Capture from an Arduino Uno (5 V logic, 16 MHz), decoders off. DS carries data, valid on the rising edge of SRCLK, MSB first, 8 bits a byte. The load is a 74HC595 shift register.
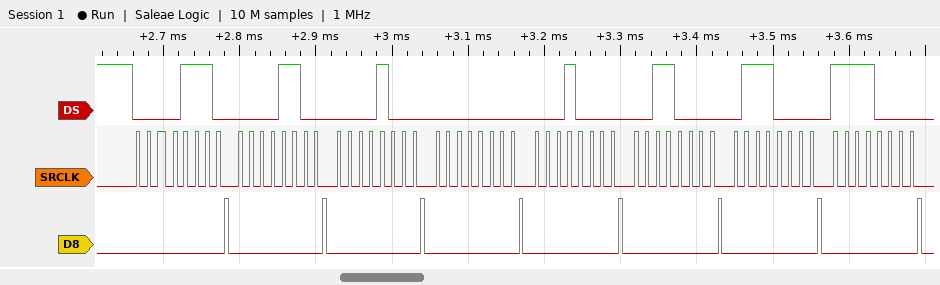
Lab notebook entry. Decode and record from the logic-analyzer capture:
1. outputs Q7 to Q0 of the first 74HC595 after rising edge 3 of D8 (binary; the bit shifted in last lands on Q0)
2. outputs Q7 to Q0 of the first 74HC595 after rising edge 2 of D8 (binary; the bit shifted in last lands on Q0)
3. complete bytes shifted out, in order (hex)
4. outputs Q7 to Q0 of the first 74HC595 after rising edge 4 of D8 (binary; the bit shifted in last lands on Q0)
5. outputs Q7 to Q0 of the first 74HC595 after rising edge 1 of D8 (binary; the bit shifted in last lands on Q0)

00001000
00001100
0x0E 0x0C 0x08 0x00 0x10 0x30 0x70 0xF0
00000000
00001110
